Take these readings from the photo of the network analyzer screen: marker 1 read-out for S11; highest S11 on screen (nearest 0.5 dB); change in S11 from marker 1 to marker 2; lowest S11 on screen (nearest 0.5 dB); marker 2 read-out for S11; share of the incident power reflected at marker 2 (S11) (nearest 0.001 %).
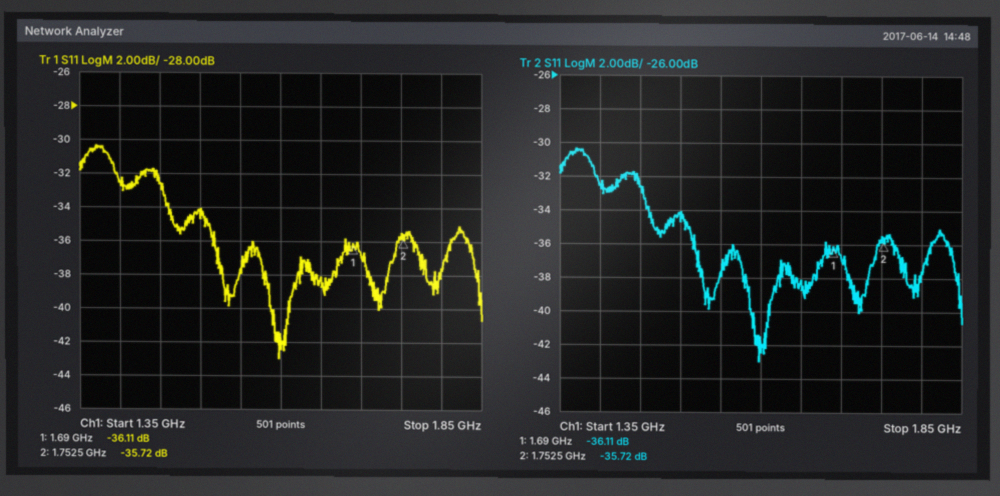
-36.11 dB
-30.5 dB
0.39 dB
-43.0 dB
-35.72 dB
0.027 %
